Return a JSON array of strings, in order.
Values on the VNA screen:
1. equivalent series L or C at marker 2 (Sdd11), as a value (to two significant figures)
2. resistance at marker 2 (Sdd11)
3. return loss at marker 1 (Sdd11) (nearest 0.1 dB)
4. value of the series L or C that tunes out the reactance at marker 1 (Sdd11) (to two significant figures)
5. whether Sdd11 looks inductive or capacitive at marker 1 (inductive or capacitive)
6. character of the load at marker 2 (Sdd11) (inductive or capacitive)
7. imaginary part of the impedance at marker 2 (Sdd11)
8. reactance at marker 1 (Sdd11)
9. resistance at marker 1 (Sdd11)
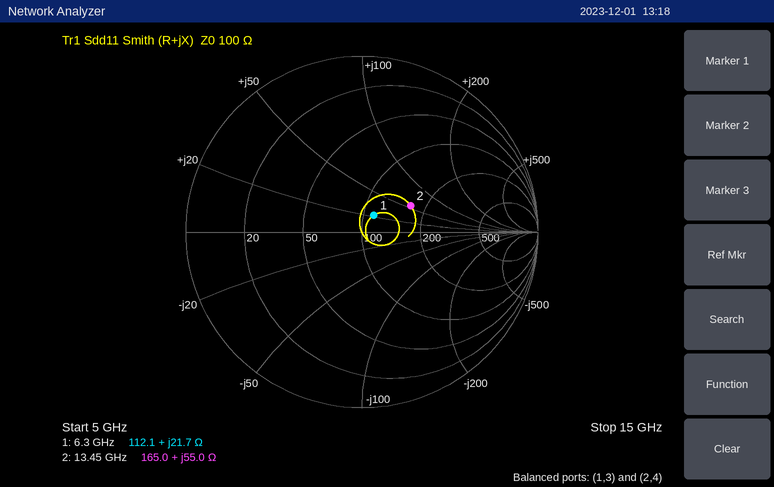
["650 pH", "165.0 Ω", "18.7 dB", "1.2 pF", "inductive", "inductive", "+55.0 Ω", "+21.7 Ω", "112.1 Ω"]
